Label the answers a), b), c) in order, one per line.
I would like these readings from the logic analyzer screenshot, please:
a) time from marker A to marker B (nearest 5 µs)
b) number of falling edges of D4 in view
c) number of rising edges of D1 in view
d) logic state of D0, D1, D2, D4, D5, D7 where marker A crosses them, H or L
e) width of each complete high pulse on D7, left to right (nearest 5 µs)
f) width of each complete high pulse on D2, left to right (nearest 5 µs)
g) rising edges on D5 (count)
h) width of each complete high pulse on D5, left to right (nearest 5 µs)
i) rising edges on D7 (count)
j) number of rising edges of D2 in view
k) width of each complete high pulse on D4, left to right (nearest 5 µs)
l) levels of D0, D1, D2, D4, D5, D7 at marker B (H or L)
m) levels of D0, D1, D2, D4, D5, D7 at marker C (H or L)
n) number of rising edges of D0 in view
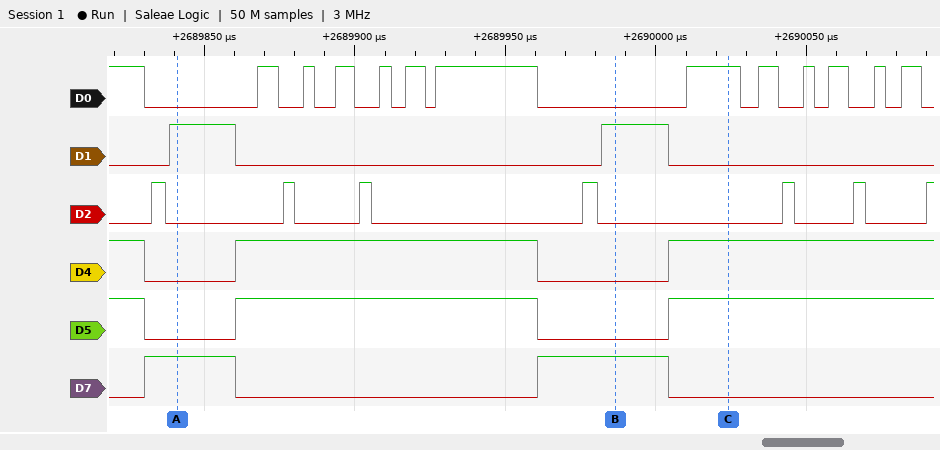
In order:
a) 145 µs
b) 2
c) 2
d) D0=L, D1=H, D2=L, D4=L, D5=L, D7=H
e) 30 µs, 45 µs
f) 5 µs, 5 µs, 5 µs, 5 µs, 5 µs, 5 µs
g) 2
h) 100 µs
i) 2
j) 7
k) 100 µs
l) D0=L, D1=H, D2=L, D4=L, D5=L, D7=H
m) D0=H, D1=L, D2=L, D4=H, D5=H, D7=L
n) 12
